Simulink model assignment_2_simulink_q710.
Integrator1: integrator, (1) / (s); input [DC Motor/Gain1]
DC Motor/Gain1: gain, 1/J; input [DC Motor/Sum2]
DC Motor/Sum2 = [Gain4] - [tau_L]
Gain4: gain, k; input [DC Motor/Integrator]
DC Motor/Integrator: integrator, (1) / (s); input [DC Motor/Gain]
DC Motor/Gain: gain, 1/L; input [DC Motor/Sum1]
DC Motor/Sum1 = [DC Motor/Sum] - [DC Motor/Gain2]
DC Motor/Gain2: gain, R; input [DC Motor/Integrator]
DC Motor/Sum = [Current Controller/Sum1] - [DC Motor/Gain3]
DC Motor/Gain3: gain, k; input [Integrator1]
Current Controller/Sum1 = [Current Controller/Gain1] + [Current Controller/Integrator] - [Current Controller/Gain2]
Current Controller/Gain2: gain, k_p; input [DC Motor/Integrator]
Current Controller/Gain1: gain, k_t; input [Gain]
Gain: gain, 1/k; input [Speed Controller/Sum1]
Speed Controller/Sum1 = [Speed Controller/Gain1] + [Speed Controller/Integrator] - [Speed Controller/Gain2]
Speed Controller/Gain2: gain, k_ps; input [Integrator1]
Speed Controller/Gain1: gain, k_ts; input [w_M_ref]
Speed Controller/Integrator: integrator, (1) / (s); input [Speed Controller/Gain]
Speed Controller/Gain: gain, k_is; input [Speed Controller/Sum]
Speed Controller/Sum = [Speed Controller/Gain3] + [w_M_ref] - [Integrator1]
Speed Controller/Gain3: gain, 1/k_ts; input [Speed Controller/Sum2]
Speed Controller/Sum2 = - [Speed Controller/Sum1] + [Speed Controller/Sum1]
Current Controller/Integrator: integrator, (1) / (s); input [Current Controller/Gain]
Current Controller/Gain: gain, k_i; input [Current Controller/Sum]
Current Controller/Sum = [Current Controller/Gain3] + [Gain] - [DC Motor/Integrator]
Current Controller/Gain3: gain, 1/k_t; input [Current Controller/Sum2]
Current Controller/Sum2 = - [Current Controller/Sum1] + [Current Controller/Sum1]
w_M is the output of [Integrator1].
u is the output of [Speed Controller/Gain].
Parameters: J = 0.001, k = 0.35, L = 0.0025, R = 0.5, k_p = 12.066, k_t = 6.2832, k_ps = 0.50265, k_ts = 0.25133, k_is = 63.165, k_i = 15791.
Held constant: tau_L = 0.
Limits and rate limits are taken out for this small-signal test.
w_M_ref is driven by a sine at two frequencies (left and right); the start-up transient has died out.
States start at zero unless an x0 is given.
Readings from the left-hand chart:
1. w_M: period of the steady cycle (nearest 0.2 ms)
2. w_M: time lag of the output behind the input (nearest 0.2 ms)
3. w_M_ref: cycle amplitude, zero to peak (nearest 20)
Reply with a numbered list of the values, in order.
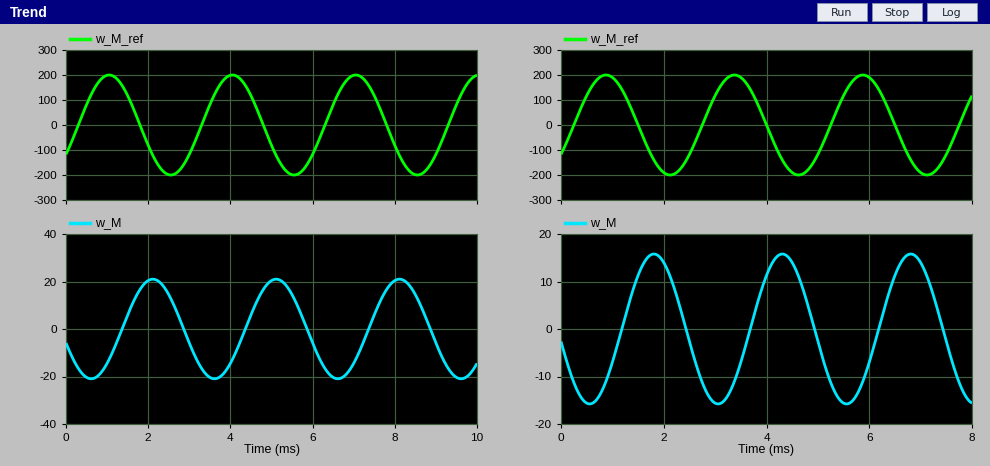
1. 3.0 ms
2. 1.0 ms
3. 200
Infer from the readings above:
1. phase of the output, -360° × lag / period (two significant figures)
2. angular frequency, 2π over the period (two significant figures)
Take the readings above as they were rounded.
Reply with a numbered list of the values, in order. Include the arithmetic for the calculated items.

1. -360 × 1 / 3 = -120°
2. 2π / 3 = 2.1 rad/ms
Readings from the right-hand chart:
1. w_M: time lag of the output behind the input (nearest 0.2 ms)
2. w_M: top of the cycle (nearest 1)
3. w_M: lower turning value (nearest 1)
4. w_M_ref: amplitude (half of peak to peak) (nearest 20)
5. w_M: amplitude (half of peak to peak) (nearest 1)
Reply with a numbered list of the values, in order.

1. 1.0 ms
2. 16
3. -16
4. 200
5. 16
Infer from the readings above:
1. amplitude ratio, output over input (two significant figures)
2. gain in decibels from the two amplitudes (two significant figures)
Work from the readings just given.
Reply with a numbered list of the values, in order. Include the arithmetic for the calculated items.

1. 16 / 200 = 0.080
2. 20 log10(16 / 200) = -22 dB
